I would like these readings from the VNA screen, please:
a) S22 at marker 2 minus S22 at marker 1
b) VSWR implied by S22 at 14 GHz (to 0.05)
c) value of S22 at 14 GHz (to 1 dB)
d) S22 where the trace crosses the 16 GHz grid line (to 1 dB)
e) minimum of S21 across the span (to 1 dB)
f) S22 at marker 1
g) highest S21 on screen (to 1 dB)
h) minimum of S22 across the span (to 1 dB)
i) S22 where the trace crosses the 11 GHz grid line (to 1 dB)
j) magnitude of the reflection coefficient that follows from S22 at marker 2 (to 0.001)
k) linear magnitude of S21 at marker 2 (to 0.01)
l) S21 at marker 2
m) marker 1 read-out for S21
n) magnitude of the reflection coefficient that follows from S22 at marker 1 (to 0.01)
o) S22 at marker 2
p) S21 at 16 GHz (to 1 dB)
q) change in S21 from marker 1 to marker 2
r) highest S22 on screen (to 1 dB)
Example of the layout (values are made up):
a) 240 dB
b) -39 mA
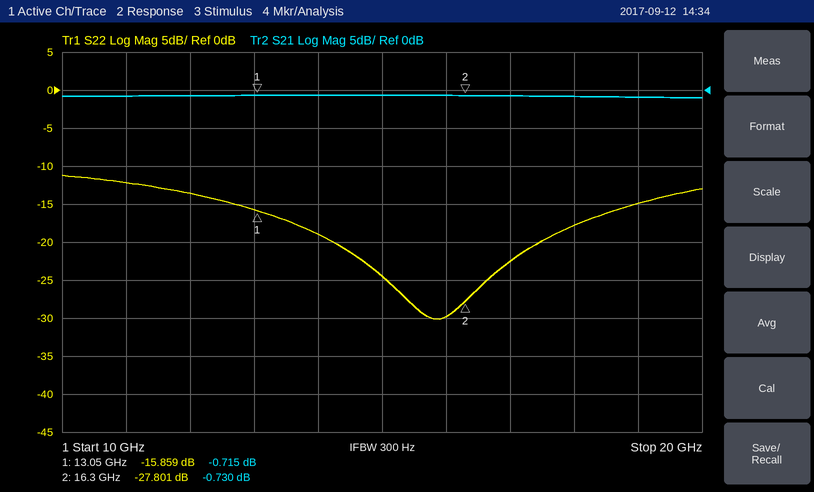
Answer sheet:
a) -11.942 dB
b) 1.25
c) -19 dB
d) -30 dB
e) -1 dB
f) -15.859 dB
g) -1 dB
h) -30 dB
i) -12 dB
j) 0.041
k) 0.92
l) -0.730 dB
m) -0.715 dB
n) 0.16
o) -27.801 dB
p) -1 dB
q) -0.015 dB
r) -11 dB
